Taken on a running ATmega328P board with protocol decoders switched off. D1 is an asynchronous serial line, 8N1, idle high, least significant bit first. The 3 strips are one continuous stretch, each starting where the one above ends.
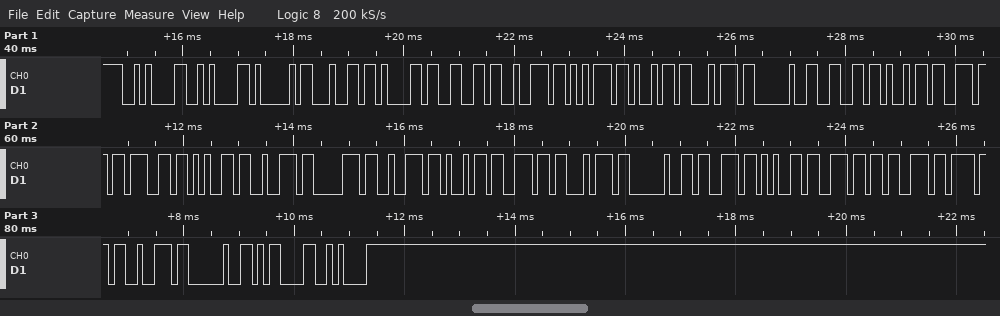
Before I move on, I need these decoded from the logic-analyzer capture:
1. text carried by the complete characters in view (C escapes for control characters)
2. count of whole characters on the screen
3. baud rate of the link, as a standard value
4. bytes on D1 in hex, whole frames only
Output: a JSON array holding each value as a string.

["\"\\n\\nAdafruit fingerprint sensor \\r\\n\"", "32", "9600 baud", "0A 0A 41 64 61 66 72 75 69 74 20 66 69 6E 67 65 72 70 72 69 6E 74 20 73 65 6E 73 6F 72 20 0D 0A"]
